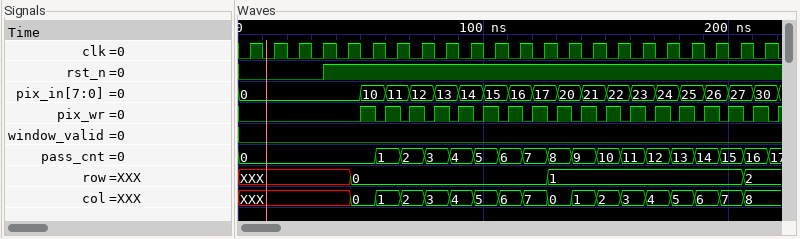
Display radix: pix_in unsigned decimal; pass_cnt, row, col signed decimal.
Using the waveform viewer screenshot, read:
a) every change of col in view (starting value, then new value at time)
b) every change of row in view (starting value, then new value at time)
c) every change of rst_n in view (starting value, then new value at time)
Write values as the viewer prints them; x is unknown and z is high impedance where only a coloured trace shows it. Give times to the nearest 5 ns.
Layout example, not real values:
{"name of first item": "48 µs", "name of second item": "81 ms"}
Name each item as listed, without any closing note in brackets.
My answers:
{"every change of col in view": "XXX, 0 at 45 ns, 1 at 55 ns, 2 at 65 ns, 3 at 75 ns, 4 at 85 ns, 5 at 95 ns, 6 at 105 ns, 7 at 115 ns, 0 at 125 ns, 1 at 135 ns, 2 at 145 ns, 3 at 155 ns, 4 at 165 ns, 5 at 175 ns, 6 at 185 ns, 7 at 195 ns, 8 at 205 ns", "every change of row in view": "XXX, 0 at 45 ns, 1 at 125 ns, 2 at 205 ns", "every change of rst_n in view": "0, 1 at 35 ns"}
